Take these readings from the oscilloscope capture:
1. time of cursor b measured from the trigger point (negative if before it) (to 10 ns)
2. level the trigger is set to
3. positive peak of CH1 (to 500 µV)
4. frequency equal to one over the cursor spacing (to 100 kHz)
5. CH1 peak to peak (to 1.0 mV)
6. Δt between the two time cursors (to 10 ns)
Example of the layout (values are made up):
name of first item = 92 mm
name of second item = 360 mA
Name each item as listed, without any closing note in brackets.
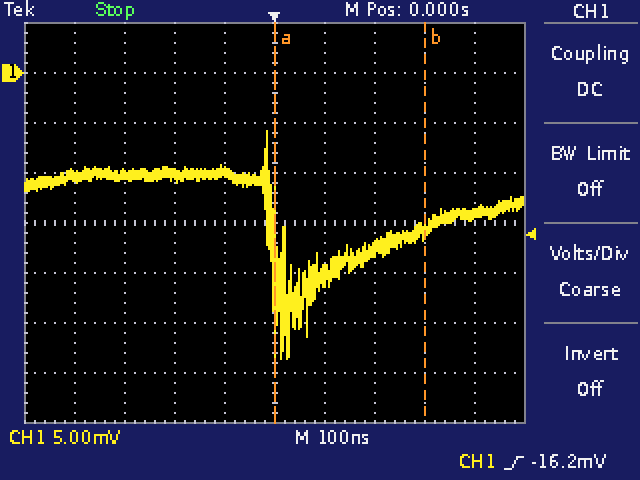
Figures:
time of cursor b measured from the trigger point (negative if before it) = +300 ns
level the trigger is set to = -16.2 mV
positive peak of CH1 = -6.0 mV
frequency equal to one over the cursor spacing = 3.3 MHz
CH1 peak to peak = 23.0 mV
Δt between the two time cursors = 300 ns
